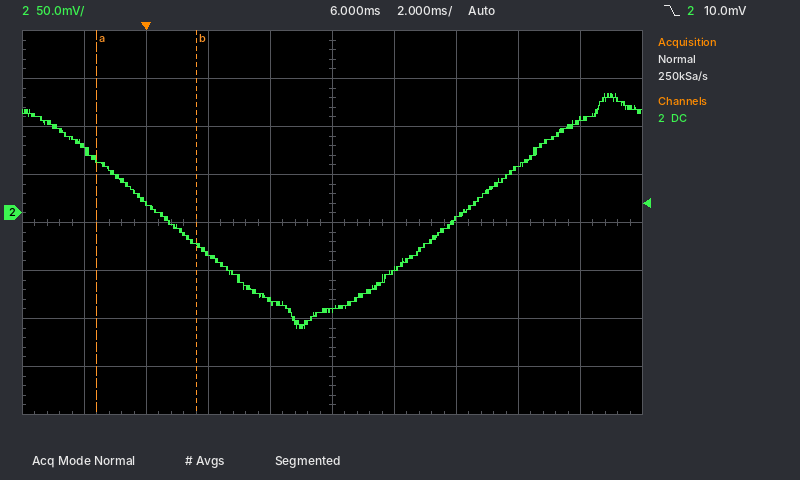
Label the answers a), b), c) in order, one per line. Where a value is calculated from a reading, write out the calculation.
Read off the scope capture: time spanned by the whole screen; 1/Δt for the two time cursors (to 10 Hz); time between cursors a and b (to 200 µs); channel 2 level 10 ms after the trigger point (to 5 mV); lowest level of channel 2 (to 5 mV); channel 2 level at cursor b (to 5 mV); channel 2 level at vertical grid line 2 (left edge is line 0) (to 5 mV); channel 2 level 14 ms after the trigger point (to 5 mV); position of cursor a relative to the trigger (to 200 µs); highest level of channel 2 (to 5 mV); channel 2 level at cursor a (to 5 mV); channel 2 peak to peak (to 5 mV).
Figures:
a) 20 ms
b) 1 / 3.2 ms ≈ 310 Hz
c) 3.2 ms
d) -10 mV
e) -120 mV
f) -35 mV
g) 10 mV
h) 95 mV
i) -1.6 ms
j) 125 mV
k) 55 mV
l) 125 mV − (-120 mV) = 245 mV
